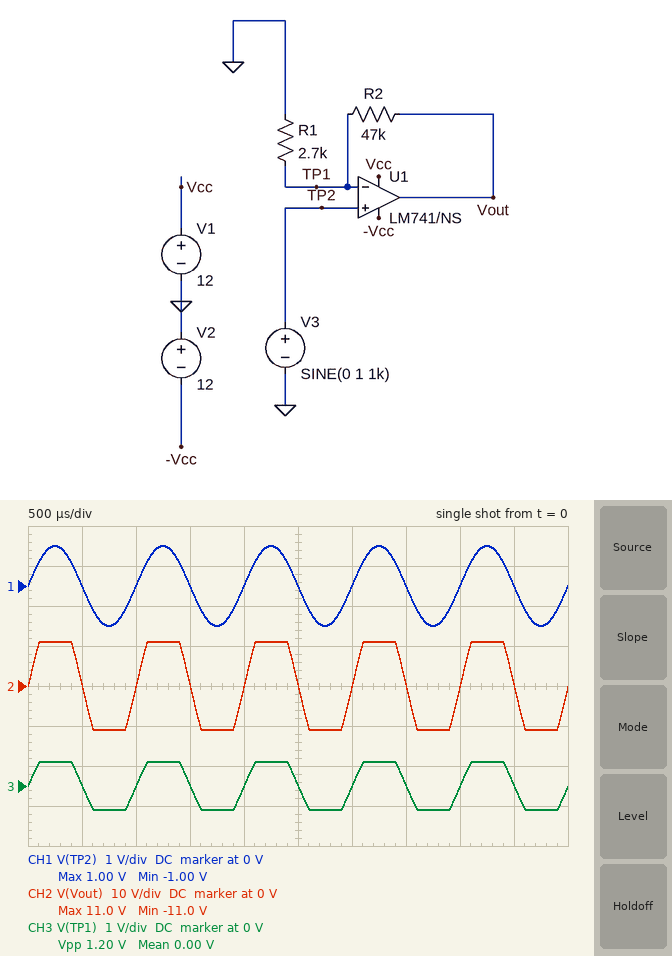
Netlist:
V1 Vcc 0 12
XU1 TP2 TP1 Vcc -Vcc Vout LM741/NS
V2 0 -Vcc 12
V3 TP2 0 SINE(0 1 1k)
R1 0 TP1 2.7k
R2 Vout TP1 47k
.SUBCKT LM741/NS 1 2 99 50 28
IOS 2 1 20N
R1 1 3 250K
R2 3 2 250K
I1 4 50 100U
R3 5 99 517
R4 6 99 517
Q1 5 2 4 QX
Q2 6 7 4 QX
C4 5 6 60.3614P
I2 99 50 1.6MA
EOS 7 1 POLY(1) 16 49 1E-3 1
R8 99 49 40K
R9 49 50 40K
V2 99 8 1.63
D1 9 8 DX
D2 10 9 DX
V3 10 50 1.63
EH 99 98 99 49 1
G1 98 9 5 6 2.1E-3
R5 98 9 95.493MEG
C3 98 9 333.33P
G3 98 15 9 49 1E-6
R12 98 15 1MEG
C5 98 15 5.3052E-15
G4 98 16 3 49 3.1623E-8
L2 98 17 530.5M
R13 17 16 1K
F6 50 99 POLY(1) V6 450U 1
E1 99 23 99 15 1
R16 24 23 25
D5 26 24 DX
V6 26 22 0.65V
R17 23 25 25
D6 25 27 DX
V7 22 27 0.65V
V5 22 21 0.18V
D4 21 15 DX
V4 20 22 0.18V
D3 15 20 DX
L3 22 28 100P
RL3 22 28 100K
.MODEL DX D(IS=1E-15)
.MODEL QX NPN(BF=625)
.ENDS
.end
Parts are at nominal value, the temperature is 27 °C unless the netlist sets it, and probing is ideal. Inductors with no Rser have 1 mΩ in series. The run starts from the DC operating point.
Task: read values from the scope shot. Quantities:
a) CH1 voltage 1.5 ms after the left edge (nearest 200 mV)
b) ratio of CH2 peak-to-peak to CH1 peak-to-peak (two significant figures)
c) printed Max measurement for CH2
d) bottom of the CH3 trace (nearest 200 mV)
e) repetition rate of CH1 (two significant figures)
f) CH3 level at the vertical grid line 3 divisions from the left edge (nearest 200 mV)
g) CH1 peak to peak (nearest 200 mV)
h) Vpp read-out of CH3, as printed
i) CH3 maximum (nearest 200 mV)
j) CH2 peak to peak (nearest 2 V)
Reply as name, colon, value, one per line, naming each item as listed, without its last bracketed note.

CH1 voltage 1.5 ms after the left edge: 0 V
ratio of CH2 peak-to-peak to CH1 peak-to-peak: 11
printed Max measurement for CH2: 11.0 V
bottom of the CH3 trace: -600 mV
repetition rate of CH1: 1.0 kHz
CH3 level at the vertical grid line 3 divisions from the left edge: 0 V
CH1 peak to peak: 2.0 V
Vpp read-out of CH3, as printed: 1.20 V
CH3 maximum: 600 mV
CH2 peak to peak: 22 V
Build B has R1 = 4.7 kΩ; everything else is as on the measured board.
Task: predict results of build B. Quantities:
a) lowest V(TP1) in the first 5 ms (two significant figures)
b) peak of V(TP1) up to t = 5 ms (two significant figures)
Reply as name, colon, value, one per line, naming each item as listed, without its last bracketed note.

lowest V(TP1) in the first 5 ms: -990 mV
peak of V(TP1) up to t = 5 ms: 990 mV
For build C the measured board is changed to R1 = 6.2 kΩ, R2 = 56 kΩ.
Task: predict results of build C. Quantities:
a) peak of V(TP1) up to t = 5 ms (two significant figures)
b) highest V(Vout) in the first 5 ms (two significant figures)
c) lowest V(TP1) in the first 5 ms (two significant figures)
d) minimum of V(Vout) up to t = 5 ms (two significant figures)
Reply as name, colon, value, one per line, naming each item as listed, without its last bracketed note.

peak of V(TP1) up to t = 5 ms: 1.0 V
highest V(Vout) in the first 5 ms: 10 V
lowest V(TP1) in the first 5 ms: -1.0 V
minimum of V(Vout) up to t = 5 ms: -10 V
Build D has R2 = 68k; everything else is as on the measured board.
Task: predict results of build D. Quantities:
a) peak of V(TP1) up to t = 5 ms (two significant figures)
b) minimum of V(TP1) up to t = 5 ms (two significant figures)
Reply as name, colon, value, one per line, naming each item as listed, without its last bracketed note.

peak of V(TP1) up to t = 5 ms: 420 mV
minimum of V(TP1) up to t = 5 ms: -420 mV
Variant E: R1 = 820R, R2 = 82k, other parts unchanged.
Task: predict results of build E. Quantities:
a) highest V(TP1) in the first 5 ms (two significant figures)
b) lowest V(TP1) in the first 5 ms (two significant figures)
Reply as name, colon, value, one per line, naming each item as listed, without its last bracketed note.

highest V(TP1) in the first 5 ms: 110 mV
lowest V(TP1) in the first 5 ms: -110 mV
